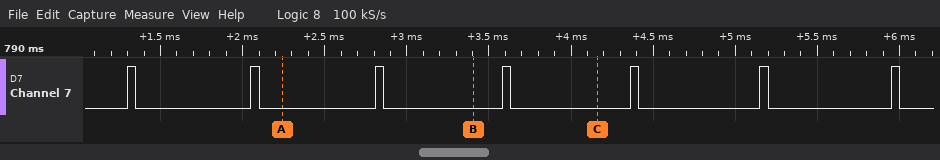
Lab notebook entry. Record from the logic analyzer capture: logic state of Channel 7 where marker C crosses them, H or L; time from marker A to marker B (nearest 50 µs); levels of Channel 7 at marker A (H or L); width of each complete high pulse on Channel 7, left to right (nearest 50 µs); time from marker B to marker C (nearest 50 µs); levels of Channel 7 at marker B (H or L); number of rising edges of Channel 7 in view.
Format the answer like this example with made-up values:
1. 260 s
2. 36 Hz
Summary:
1. Channel 7=L
2. 1150 µs
3. Channel 7=L
4. 50 µs, 50 µs, 50 µs, 50 µs, 50 µs, 50 µs, 50 µs
5. 750 µs
6. Channel 7=L
7. 7
